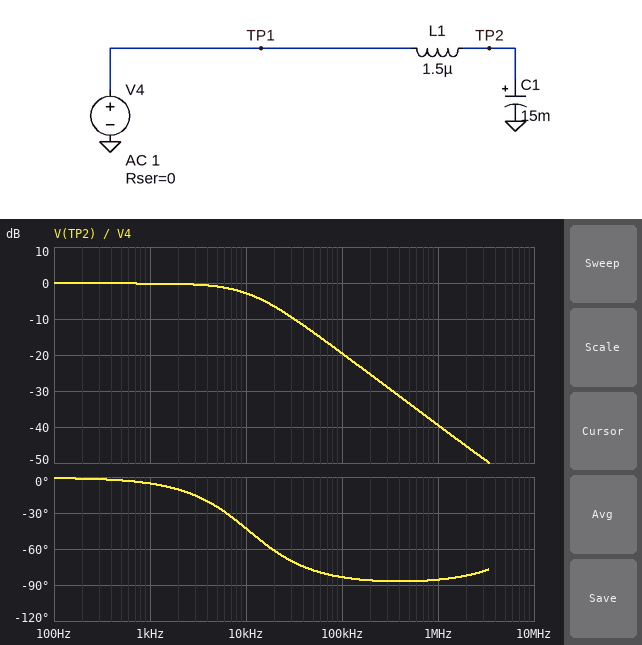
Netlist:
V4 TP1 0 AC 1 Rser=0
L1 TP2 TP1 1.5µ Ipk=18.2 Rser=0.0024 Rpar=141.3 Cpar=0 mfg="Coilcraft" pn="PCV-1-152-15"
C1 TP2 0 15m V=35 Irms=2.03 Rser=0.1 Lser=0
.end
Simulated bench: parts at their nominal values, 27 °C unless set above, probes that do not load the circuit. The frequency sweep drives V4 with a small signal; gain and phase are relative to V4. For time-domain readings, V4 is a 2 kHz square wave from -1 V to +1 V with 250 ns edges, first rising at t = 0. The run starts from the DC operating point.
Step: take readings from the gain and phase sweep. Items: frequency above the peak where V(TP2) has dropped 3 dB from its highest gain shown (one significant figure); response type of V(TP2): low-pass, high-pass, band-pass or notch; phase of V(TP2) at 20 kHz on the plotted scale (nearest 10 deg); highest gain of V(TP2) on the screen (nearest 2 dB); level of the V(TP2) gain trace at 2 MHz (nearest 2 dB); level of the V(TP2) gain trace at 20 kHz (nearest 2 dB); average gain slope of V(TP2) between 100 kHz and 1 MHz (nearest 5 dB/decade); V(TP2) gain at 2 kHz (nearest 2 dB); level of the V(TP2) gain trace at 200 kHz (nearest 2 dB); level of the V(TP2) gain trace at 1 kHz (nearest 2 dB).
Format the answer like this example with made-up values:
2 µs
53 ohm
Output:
10 kHz
low-pass
-60 deg
0 dB
-46 dB
-6 dB
-20 dB/decade
0 dB
-26 dB
0 dB
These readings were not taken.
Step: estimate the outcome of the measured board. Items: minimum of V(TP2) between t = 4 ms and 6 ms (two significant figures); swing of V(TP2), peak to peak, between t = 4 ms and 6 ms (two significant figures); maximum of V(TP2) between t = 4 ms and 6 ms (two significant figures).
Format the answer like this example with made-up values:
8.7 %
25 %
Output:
-990 mV
2.0 V
990 mV
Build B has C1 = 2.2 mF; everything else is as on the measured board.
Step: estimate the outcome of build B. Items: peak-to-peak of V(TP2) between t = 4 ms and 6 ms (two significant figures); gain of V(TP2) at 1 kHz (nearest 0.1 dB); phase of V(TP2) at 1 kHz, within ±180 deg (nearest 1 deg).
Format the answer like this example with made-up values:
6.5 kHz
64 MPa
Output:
2.1 V
0.2 dB
-4 deg
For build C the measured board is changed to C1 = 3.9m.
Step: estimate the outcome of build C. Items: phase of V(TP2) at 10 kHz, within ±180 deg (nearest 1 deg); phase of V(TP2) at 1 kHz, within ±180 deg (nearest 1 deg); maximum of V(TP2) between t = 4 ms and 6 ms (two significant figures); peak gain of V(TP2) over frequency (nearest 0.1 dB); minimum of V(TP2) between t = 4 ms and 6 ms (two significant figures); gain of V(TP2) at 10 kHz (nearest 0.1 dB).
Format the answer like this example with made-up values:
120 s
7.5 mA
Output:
-44 deg
-5 deg
1.0 V
0.1 dB
-1.0 V
-2.7 dB
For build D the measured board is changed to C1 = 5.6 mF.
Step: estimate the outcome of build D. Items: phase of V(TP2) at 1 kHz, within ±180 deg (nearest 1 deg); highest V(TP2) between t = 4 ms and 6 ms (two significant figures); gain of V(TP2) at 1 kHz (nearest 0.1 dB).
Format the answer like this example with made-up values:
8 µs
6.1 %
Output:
-5 deg
1.0 V
0 dB
